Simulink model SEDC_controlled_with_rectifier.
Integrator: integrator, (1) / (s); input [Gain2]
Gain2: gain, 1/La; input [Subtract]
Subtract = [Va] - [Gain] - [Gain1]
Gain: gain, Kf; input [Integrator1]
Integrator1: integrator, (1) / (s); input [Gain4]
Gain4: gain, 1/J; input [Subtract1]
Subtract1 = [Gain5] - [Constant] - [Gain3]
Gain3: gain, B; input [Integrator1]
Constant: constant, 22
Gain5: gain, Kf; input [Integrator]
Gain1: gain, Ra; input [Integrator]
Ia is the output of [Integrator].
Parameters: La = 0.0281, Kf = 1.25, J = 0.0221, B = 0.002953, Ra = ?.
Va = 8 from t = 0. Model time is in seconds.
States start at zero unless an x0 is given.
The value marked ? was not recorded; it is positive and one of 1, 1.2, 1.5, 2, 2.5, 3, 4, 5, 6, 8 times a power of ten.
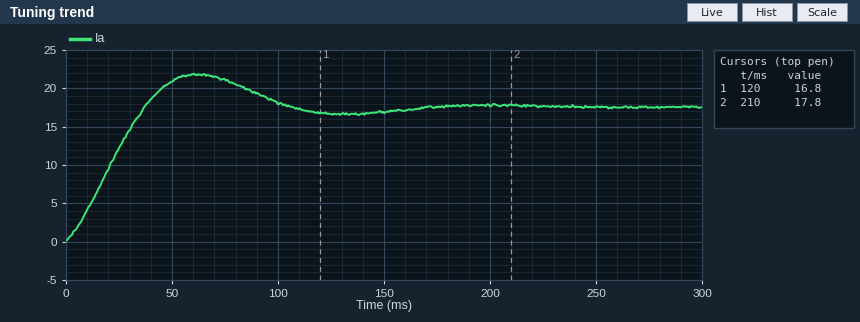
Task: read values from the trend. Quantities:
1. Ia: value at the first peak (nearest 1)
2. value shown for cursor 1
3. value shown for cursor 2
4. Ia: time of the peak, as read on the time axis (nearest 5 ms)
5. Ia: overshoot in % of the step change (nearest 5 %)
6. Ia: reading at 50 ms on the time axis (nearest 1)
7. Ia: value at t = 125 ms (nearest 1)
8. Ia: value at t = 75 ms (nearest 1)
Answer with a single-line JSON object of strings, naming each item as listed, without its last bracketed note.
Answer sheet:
{"Ia: value at the first peak": "22", "value shown for cursor 1": "16.8", "value shown for cursor 2": "17.8", "Ia: time of the peak, as read on the time axis": "60 ms", "Ia: overshoot in % of the step change": "25 %", "Ia: reading at 50 ms on the time axis": "21", "Ia: value at t = 125 ms": "17", "Ia: value at t = 75 ms": "21"}
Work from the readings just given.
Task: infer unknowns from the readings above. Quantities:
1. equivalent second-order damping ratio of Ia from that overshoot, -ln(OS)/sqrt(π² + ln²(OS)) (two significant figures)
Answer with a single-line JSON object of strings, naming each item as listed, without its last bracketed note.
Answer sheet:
{"equivalent second-order damping ratio of Ia from that overshoot, -ln(OS)/sqrt(π² + ln²(OS))": "0.40"}
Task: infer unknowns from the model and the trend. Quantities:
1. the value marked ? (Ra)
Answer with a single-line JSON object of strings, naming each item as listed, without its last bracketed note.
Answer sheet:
{"the value marked ?": "1.2"}
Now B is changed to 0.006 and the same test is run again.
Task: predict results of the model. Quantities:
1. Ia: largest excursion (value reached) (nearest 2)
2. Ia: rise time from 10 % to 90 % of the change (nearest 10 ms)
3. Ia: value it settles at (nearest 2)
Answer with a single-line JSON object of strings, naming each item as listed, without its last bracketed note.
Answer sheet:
{"Ia: largest excursion (value reached)": "22", "Ia: rise time from 10 % to 90 % of the change": "30 ms", "Ia: value it settles at": "18"}
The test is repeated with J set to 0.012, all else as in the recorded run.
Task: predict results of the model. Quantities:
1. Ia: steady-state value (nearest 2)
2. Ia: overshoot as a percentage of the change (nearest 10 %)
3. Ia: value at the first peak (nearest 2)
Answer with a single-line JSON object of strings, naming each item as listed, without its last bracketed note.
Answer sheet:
{"Ia: steady-state value": "18", "Ia: overshoot as a percentage of the change": "40 %", "Ia: value at the first peak": "24"}
